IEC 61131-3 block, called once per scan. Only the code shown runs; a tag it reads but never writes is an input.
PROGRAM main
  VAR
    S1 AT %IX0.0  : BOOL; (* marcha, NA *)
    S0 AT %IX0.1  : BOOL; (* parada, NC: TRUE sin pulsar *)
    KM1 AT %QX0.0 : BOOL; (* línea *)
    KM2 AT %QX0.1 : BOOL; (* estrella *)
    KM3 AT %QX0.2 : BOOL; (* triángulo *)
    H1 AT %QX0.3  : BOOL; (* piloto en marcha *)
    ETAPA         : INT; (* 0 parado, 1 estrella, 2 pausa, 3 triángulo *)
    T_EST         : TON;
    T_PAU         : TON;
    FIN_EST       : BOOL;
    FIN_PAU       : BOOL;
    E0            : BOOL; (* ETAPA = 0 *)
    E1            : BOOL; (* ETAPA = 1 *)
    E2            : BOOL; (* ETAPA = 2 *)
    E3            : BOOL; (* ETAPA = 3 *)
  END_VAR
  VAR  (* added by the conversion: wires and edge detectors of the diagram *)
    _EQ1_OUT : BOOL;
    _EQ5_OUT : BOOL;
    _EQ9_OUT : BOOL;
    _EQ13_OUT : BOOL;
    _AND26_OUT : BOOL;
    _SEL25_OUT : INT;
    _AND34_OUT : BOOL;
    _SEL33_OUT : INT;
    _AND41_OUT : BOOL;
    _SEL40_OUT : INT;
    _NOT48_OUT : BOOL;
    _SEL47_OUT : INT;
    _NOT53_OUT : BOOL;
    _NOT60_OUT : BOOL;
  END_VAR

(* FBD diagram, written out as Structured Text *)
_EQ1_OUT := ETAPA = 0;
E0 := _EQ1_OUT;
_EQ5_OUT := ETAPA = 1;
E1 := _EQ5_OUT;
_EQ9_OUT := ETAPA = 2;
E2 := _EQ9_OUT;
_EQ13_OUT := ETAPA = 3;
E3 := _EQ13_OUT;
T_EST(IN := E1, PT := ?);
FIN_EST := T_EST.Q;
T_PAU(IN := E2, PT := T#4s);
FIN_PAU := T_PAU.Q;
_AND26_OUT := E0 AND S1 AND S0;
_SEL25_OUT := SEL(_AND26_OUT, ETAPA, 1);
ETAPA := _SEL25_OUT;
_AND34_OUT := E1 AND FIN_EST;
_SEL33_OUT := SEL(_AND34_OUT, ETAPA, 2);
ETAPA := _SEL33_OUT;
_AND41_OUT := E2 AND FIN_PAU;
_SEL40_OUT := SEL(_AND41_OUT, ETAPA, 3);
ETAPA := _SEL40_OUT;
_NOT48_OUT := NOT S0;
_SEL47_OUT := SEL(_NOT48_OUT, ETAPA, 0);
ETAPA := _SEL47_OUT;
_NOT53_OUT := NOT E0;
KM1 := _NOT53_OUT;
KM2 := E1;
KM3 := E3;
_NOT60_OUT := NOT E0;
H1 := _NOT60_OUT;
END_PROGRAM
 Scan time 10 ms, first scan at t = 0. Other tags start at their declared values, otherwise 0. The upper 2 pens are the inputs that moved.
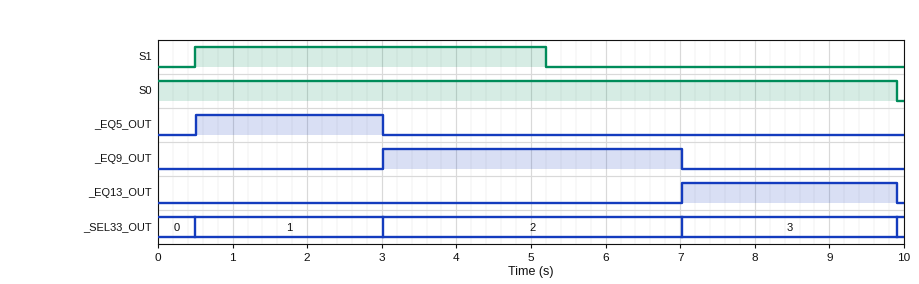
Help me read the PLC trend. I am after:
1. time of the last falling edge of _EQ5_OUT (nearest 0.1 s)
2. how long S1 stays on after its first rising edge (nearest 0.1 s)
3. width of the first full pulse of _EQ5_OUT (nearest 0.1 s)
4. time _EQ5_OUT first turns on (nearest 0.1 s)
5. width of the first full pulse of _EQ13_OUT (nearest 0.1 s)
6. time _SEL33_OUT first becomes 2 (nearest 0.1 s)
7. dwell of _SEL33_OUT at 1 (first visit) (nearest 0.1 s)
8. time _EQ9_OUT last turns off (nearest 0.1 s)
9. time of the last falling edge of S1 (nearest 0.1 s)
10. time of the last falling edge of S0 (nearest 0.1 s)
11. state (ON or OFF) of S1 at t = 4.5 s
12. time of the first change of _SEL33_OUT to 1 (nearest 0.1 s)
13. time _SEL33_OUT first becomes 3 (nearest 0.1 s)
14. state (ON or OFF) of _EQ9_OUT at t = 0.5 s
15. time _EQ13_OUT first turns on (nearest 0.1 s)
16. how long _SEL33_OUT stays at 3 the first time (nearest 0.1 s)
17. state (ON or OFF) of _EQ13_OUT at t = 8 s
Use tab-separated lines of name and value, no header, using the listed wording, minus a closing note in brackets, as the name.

time of the last falling edge of _EQ5_OUT	3.0 s
how long S1 stays on after its first rising edge	4.7 s
width of the first full pulse of _EQ5_OUT	2.5 s
time _EQ5_OUT first turns on	0.5 s
width of the first full pulse of _EQ13_OUT	2.9 s
time _SEL33_OUT first becomes 2	3.0 s
dwell of _SEL33_OUT at 1 (first visit)	2.5 s
time _EQ9_OUT last turns off	7.0 s
time of the last falling edge of S1	5.2 s
time of the last falling edge of S0	9.9 s
state (ON or OFF) of S1 at t = 4.5 s	ON
time of the first change of _SEL33_OUT to 1	0.5 s
time _SEL33_OUT first becomes 3	7.0 s
state (ON or OFF) of _EQ9_OUT at t = 0.5 s	OFF
time _EQ13_OUT first turns on	7.0 s
how long _SEL33_OUT stays at 3 the first time	2.9 s
state (ON or OFF) of _EQ13_OUT at t = 8 s	ON
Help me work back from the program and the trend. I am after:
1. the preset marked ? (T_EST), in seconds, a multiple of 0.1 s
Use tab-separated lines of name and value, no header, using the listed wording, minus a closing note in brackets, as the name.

the preset marked ? (T_EST), in seconds, a multiple of 0.1 s	2.5 s
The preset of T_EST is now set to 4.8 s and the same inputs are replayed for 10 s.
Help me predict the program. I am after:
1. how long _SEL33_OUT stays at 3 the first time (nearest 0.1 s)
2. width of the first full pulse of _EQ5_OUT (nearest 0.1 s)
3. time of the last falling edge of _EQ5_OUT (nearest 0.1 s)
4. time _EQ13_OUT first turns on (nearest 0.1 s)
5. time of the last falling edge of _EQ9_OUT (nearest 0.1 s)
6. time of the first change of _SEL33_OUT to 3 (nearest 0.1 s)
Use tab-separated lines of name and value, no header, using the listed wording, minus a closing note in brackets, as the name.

how long _SEL33_OUT stays at 3 the first time	0.6 s
width of the first full pulse of _EQ5_OUT	4.8 s
time of the last falling edge of _EQ5_OUT	5.3 s
time _EQ13_OUT first turns on	9.3 s
time of the last falling edge of _EQ9_OUT	9.3 s
time of the first change of _SEL33_OUT to 3	9.3 s
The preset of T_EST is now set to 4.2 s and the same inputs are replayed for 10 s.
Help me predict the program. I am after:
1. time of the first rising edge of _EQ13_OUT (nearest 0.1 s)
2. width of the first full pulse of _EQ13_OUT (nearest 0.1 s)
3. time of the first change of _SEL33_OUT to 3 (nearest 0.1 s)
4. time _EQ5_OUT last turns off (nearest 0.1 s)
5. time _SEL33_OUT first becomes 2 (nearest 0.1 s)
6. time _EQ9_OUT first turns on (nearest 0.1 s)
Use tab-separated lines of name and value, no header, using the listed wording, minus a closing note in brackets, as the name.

time of the first rising edge of _EQ13_OUT	8.7 s
width of the first full pulse of _EQ13_OUT	1.2 s
time of the first change of _SEL33_OUT to 3	8.7 s
time _EQ5_OUT last turns off	4.7 s
time _SEL33_OUT first becomes 2	4.7 s
time _EQ9_OUT first turns on	4.7 s
